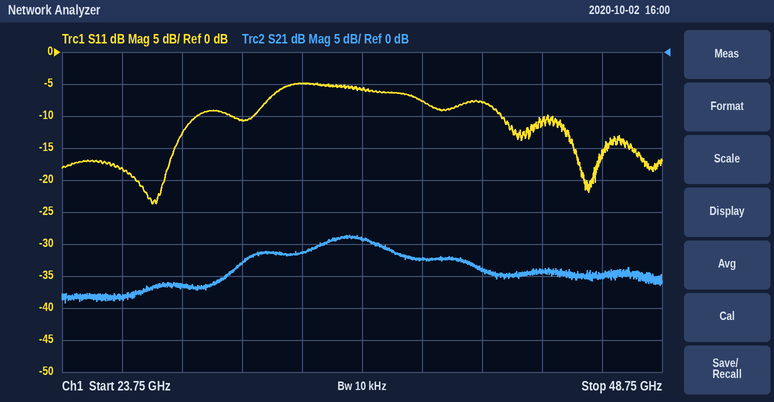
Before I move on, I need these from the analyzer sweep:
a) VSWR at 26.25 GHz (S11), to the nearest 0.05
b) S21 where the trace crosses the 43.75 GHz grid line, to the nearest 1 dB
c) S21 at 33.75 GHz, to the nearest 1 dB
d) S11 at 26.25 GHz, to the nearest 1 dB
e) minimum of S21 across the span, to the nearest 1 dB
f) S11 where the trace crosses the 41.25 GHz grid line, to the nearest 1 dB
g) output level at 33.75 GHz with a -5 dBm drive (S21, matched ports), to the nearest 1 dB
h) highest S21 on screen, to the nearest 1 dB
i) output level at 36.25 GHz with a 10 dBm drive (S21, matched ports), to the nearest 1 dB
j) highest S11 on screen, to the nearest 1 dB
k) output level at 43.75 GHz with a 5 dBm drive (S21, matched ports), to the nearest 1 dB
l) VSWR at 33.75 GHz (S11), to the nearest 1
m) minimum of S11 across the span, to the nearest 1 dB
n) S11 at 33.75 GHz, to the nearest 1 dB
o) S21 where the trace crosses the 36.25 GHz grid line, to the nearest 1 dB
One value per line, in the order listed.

1.30
-34 dB
-31 dB
-18 dB
-39 dB
-8 dB
-36 dBm
-29 dB
-19 dBm
-5 dB
-29 dBm
4
-24 dB
-5 dB
-29 dB
